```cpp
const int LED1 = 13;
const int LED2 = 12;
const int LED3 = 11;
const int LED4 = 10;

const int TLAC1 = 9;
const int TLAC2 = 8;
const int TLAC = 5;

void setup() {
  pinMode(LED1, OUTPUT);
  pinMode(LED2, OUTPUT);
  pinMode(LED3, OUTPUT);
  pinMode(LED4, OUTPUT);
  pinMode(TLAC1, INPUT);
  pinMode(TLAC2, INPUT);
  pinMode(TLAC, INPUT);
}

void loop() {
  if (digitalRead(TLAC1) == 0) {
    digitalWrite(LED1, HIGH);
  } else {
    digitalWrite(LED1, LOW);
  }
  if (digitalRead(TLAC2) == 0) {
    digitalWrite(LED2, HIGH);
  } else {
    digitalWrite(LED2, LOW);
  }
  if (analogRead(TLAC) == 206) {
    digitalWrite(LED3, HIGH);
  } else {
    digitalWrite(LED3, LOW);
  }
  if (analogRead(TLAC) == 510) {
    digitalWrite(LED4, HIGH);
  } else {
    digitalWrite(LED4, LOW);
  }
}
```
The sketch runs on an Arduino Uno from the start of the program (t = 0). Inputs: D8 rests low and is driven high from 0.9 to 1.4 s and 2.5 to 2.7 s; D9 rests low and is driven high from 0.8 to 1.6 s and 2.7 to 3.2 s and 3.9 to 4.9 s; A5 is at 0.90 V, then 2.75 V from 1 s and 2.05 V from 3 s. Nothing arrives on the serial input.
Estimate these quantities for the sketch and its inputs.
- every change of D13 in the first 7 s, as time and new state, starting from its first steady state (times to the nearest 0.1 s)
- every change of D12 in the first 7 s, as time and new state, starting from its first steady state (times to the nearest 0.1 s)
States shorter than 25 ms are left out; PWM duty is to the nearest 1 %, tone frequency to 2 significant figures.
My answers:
0 s high; 0.8 s low; 1.6 s high; 2.7 s low; 3.2 s high; 3.9 s low; 4.9 s high
0 s high; 0.9 s low; 1.4 s high; 2.5 s low; 2.7 s high
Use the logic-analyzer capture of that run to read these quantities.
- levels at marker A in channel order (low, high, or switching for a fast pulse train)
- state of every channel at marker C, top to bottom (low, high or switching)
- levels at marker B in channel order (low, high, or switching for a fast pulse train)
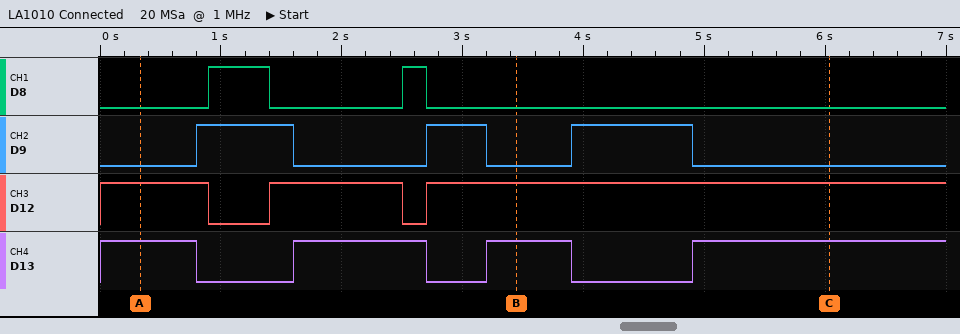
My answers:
D8 low, D9 low, D12 high, D13 high
D8 low, D9 low, D12 high, D13 high
D8 low, D9 low, D12 high, D13 high
